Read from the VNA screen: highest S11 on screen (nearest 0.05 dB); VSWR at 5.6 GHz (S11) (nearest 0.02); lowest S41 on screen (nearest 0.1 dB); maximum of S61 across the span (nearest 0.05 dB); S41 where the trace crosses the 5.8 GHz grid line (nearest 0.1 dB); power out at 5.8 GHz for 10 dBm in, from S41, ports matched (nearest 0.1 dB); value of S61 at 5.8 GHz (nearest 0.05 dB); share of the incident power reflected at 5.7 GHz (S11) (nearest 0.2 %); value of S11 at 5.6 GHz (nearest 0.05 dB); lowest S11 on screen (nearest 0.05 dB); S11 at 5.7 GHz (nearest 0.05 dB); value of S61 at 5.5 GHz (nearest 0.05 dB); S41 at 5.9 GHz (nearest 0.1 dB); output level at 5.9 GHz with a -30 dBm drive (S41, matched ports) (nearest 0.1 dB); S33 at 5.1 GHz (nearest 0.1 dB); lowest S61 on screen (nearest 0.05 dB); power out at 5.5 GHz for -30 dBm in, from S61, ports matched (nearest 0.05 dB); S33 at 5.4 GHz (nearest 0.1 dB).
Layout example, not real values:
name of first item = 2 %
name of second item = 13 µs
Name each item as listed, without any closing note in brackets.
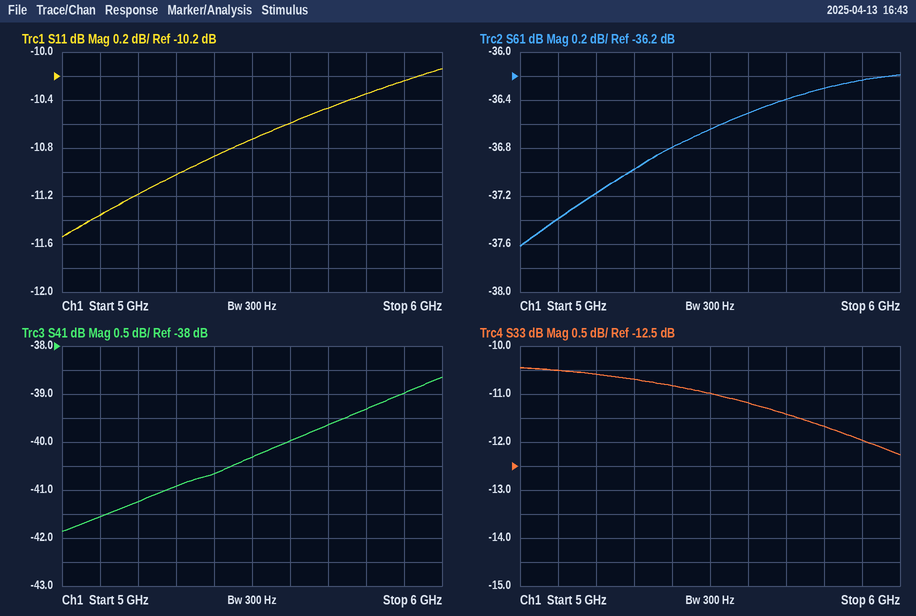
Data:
highest S11 on screen = -10.15 dB
VSWR at 5.6 GHz (S11) = 1.84
lowest S41 on screen = -41.9 dB
maximum of S61 across the span = -36.20 dB
S41 where the trace crosses the 5.8 GHz grid line = -39.3 dB
power out at 5.8 GHz for 10 dBm in, from S41, ports matched = -29.3 dBm
value of S61 at 5.8 GHz = -36.30 dB
share of the incident power reflected at 5.7 GHz (S11) = 9.0 %
value of S11 at 5.6 GHz = -10.60 dB
lowest S11 on screen = -11.55 dB
S11 at 5.7 GHz = -10.45 dB
value of S61 at 5.5 GHz = -36.65 dB
S41 at 5.9 GHz = -39.0 dB
output level at 5.9 GHz with a -30 dBm drive (S41, matched ports) = -69.0 dBm
S33 at 5.1 GHz = -10.5 dB
lowest S61 on screen = -37.60 dB
power out at 5.5 GHz for -30 dBm in, from S61, ports matched = -66.65 dBm
S33 at 5.4 GHz = -10.8 dB
